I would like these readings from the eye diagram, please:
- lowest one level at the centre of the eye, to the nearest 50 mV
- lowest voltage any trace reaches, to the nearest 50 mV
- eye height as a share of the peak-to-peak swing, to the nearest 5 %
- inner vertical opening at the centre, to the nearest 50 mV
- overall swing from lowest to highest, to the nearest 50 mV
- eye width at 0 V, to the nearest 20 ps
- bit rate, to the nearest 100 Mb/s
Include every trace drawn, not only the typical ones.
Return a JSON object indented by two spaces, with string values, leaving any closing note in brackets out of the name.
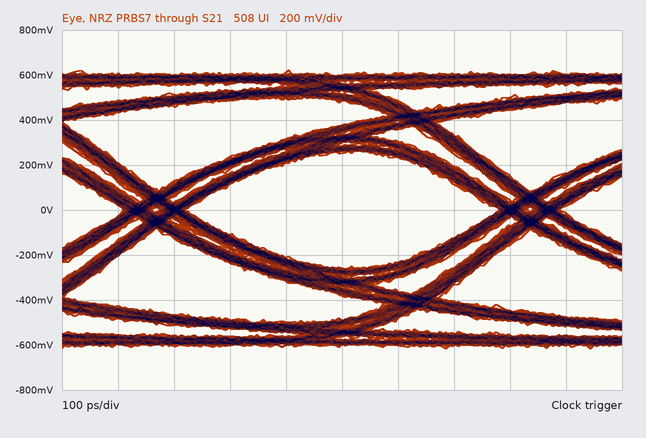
{
  "lowest one level at the centre of the eye, to the nearest 50 mV": "250 mV",
  "lowest voltage any trace reaches, to the nearest 50 mV": "-600 mV",
  "eye height as a share of the peak-to-peak swing, to the nearest 5 %": "40 %",
  "inner vertical opening at the centre, to the nearest 50 mV": "500 mV",
  "overall swing from lowest to highest, to the nearest 50 mV": "1.25 V",
  "eye width at 0 V, to the nearest 20 ps": "560 ps",
  "bit rate, to the nearest 100 Mb/s": "1.5 Gb/s"
}
